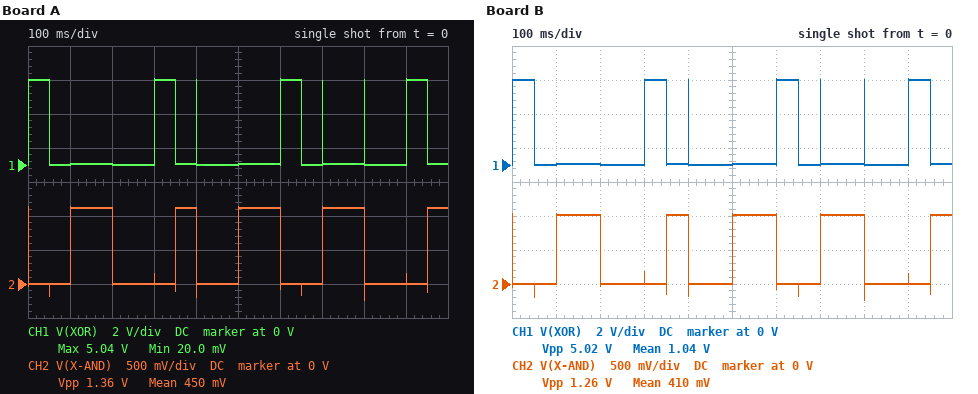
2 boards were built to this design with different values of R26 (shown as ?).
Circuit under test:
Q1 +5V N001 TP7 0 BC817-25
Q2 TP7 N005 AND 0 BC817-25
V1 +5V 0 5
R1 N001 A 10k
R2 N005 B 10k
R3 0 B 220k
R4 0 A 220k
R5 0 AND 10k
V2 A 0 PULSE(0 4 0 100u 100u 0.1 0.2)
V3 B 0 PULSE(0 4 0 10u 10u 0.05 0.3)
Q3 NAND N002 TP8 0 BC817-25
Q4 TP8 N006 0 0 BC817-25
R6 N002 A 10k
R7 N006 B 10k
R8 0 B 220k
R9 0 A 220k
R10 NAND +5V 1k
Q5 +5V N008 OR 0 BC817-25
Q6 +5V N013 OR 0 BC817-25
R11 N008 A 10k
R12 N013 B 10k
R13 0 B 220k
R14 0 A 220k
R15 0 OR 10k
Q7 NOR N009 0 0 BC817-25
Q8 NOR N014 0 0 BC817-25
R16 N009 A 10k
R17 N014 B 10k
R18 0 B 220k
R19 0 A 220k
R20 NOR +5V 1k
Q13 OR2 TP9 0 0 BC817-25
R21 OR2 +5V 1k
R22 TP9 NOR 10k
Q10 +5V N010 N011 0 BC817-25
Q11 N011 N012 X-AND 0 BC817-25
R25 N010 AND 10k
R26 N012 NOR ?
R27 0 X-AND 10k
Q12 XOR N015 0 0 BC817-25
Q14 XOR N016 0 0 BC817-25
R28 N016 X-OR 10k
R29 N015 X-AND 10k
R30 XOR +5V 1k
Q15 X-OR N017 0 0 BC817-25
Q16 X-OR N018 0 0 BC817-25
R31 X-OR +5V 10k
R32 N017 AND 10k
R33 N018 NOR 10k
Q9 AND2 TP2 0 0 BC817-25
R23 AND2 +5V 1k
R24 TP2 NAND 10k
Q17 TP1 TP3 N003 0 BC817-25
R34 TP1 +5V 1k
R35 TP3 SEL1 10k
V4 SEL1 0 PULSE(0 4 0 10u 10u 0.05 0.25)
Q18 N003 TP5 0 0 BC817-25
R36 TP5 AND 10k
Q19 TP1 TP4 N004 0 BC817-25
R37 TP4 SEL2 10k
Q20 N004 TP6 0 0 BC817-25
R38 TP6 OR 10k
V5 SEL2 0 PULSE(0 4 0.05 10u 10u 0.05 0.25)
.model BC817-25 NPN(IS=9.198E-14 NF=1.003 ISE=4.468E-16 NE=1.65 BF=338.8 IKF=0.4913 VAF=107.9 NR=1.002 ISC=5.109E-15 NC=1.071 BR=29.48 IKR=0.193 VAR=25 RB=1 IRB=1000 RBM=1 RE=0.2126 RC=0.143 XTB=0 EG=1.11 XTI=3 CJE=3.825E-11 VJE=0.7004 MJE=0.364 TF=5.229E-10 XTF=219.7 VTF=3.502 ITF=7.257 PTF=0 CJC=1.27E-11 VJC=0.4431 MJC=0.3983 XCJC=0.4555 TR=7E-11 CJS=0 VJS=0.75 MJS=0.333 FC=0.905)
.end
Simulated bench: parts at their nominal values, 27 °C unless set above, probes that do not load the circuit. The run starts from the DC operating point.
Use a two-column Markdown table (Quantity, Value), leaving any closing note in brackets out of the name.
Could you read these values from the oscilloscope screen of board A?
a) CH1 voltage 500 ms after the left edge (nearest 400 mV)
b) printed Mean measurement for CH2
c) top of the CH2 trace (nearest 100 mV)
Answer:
| Quantity | Value |
|---|---|
| CH1 voltage 500 ms after the left edge | 0 V |
| printed Mean measurement for CH2 | 450 mV |
| top of the CH2 trace | 1.1 V |
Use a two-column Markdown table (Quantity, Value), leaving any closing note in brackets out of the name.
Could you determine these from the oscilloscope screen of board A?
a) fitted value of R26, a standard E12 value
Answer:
| Quantity | Value |
|---|---|
| fitted value of R26, a standard E12 value | 15 kΩ |
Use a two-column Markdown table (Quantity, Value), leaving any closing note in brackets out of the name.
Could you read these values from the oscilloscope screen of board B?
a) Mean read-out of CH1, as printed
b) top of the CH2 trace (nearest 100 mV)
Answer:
| Quantity | Value |
|---|---|
| Mean read-out of CH1, as printed | 1.04 V |
| top of the CH2 trace | 1.0 V |
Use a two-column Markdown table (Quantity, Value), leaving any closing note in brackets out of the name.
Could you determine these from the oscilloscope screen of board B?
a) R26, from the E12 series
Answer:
| Quantity | Value |
|---|---|
| R26, from the E12 series | 18 kΩ |
